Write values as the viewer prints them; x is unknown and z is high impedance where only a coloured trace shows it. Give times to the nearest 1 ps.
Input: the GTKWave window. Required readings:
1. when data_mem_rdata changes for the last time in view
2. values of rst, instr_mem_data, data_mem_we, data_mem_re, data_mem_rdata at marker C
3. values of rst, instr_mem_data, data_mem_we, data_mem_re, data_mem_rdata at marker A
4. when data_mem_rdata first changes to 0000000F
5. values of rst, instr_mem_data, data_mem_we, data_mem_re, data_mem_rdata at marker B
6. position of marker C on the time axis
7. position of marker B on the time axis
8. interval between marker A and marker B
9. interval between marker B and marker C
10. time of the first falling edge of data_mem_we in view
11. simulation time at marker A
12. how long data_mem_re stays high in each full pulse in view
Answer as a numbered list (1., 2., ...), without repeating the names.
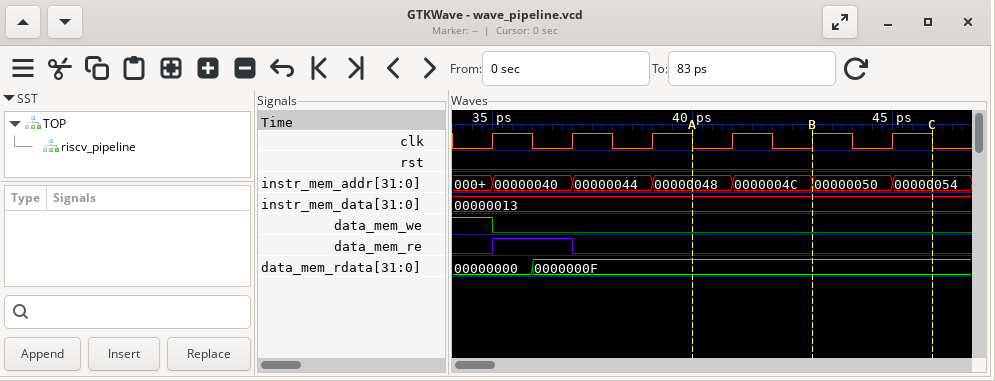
1. 36 ps
2. rst=0, instr_mem_data=00000013, data_mem_we=0, data_mem_re=0, data_mem_rdata=0000000F
3. rst=0, instr_mem_data=00000013, data_mem_we=0, data_mem_re=0, data_mem_rdata=0000000F
4. 36 ps
5. rst=0, instr_mem_data=00000013, data_mem_we=0, data_mem_re=0, data_mem_rdata=0000000F
6. 46 ps
7. 43 ps
8. 3 ps
9. 3 ps
10. 35 ps
11. 40 ps
12. 2 ps
